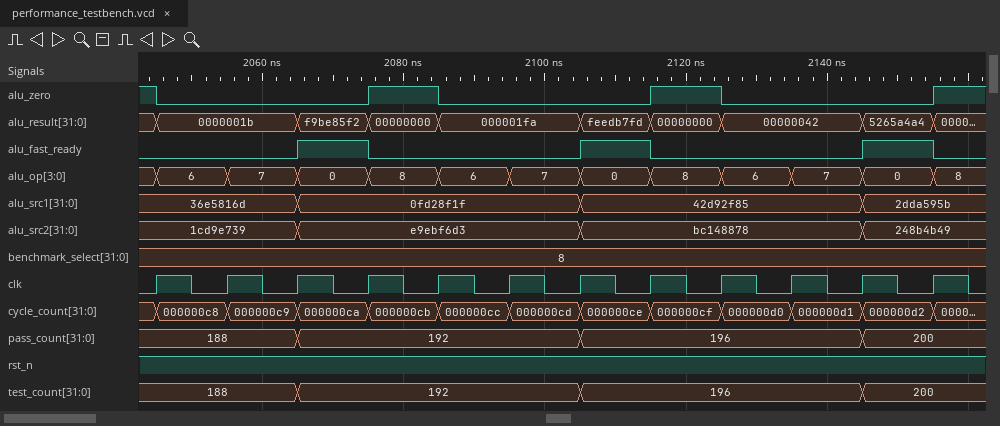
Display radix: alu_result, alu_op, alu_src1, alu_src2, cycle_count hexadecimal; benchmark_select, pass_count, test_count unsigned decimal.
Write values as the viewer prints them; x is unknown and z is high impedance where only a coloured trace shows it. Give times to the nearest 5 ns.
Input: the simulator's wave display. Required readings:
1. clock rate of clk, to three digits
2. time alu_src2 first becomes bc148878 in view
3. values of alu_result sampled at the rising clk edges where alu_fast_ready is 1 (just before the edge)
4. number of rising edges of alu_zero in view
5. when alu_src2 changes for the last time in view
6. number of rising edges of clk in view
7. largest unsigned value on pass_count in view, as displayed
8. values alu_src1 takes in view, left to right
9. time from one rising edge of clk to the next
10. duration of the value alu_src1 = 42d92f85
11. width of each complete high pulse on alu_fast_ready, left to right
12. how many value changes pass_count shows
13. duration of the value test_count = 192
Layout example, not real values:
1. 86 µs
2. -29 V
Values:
1. 100 MHz
2. 2105 ns
3. f9be85f2, feedb7fd, 5265a4a4
4. 3
5. 2145 ns
6. 12
7. 200
8. 36e5816d, 0fd28f1f, 42d92f85, 2dda595b
9. 10 ns
10. 40 ns
11. 10 ns, 10 ns, 10 ns
12. 3
13. 40 ns
